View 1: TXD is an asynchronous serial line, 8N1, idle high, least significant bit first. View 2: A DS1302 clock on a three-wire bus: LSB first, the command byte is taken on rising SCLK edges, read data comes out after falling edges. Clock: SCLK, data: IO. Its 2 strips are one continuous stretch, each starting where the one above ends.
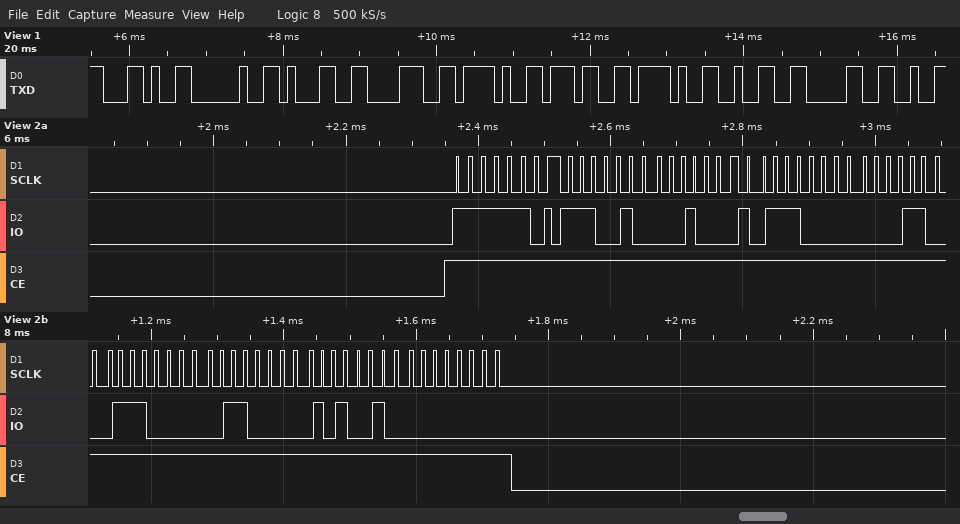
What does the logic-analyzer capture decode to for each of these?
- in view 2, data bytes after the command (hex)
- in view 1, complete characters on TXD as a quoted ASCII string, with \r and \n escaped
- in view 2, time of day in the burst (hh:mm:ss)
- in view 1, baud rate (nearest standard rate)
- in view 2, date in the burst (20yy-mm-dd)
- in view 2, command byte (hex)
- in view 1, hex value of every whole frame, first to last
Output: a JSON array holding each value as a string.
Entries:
["27 44 07 18 07 06 25 00", "\", 18/7/20\"", "07:44:27", "9600 baud", "2025-07-18", "0xBF", "2C 20 31 38 2F 37 2F 32 30"]
